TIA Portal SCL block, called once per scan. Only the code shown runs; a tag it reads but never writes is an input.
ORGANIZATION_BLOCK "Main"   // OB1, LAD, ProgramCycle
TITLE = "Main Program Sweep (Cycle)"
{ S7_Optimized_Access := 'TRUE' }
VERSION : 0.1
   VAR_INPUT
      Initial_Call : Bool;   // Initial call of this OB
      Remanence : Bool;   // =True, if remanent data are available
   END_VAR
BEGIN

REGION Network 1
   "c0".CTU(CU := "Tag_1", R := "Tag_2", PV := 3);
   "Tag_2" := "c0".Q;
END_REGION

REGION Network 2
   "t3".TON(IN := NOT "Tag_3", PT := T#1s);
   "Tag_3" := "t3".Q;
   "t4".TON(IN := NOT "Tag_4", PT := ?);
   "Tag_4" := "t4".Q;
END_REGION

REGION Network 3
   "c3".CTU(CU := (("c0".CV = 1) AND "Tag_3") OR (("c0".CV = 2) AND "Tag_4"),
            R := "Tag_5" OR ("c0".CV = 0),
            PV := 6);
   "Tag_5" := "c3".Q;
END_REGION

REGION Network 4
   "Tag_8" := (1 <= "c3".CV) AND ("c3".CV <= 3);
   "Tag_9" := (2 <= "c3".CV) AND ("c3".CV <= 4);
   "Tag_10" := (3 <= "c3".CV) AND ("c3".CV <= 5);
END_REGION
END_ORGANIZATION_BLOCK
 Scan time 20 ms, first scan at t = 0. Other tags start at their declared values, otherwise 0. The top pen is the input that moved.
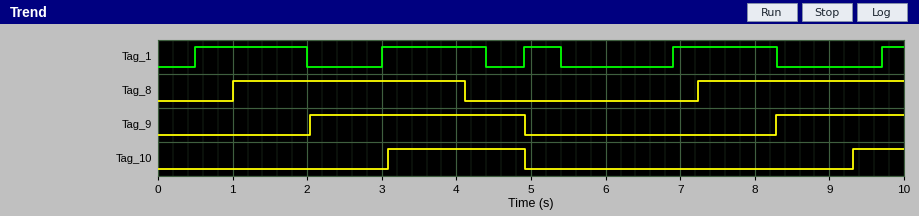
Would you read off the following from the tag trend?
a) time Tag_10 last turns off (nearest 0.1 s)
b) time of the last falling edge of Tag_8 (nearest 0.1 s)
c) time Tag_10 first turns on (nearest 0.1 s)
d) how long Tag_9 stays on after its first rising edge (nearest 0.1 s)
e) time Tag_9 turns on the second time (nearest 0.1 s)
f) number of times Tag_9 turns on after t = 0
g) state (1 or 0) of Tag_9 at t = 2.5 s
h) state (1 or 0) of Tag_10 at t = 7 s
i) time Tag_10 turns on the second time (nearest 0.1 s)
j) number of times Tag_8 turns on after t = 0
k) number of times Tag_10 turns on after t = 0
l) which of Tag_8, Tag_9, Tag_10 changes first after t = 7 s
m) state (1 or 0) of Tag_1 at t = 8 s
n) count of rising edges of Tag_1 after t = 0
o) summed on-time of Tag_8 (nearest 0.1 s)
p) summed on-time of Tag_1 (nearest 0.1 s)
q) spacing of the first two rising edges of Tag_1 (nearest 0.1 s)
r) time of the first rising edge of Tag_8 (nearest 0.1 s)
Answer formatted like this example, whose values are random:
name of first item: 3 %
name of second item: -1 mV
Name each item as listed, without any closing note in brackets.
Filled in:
time Tag_10 last turns off: 4.9 s
time of the last falling edge of Tag_8: 4.1 s
time Tag_10 first turns on: 3.1 s
how long Tag_9 stays on after its first rising edge: 2.9 s
time Tag_9 turns on the second time: 8.3 s
number of times Tag_9 turns on after t = 0: 2
state (1 or 0) of Tag_9 at t = 2.5 s: 1
state (1 or 0) of Tag_10 at t = 7 s: 0
time Tag_10 turns on the second time: 9.3 s
number of times Tag_8 turns on after t = 0: 2
number of times Tag_10 turns on after t = 0: 2
which of Tag_8, Tag_9, Tag_10 changes first after t = 7 s: Tag_8
state (1 or 0) of Tag_1 at t = 8 s: 1
count of rising edges of Tag_1 after t = 0: 5
summed on-time of Tag_8: 5.9 s
summed on-time of Tag_1: 5.1 s
spacing of the first two rising edges of Tag_1: 2.5 s
time of the first rising edge of Tag_8: 1.0 s
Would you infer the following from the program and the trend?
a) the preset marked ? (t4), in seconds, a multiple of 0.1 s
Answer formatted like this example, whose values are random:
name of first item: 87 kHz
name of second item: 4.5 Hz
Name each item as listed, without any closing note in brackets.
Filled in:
the preset marked ? (t4), in seconds, a multiple of 0.1 s: 1.0 s
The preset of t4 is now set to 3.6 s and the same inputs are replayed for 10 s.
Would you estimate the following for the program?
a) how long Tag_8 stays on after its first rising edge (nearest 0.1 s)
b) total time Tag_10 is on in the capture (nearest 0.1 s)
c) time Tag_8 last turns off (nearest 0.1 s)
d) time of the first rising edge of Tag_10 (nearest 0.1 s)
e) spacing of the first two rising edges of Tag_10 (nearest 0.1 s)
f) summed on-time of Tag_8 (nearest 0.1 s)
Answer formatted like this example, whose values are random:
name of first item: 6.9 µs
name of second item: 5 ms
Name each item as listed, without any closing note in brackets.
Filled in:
how long Tag_8 stays on after its first rising edge: 3.9 s
total time Tag_10 is on in the capture: 2.0 s
time Tag_8 last turns off: 4.9 s
time of the first rising edge of Tag_10: 3.6 s
spacing of the first two rising edges of Tag_10: 5.7 s
summed on-time of Tag_8: 6.7 s
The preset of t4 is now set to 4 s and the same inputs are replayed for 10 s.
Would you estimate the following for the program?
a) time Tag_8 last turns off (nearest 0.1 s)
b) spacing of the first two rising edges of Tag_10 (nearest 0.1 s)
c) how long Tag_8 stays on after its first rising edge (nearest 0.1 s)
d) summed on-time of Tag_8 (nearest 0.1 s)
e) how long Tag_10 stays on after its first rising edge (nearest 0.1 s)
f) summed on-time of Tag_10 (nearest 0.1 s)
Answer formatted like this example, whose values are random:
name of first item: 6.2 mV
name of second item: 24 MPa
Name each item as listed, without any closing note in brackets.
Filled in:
time Tag_8 last turns off: 4.9 s
spacing of the first two rising edges of Tag_10: 5.3 s
how long Tag_8 stays on after its first rising edge: 3.9 s
summed on-time of Tag_8: 6.7 s
how long Tag_10 stays on after its first rising edge: 0.9 s
summed on-time of Tag_10: 1.6 s
